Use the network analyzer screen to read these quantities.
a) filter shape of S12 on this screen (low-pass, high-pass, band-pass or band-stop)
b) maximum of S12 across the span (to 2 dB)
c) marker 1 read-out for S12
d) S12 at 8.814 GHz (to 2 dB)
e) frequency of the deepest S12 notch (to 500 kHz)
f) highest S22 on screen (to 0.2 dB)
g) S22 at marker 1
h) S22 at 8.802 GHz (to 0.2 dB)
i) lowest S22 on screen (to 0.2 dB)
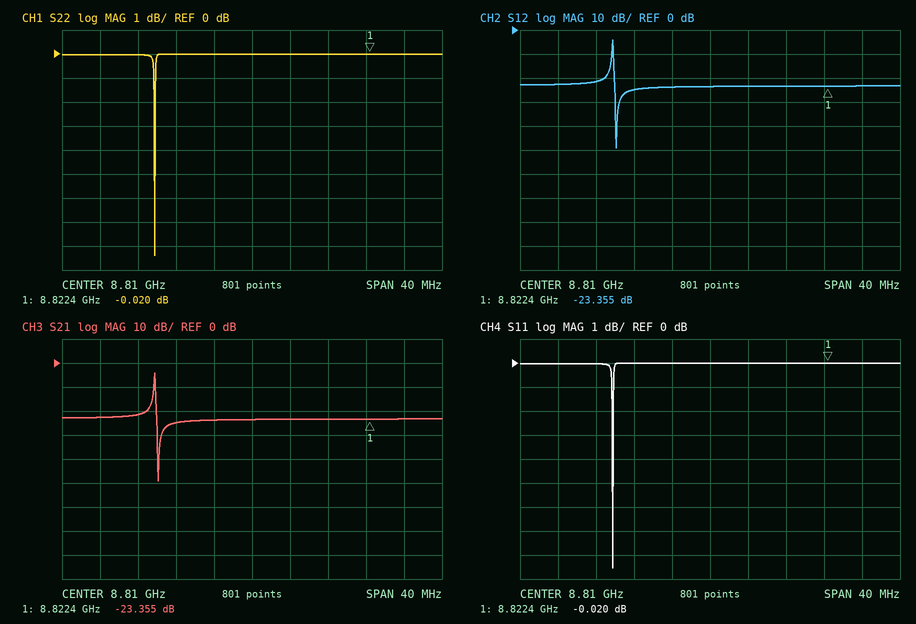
band-pass
-4 dB
-23.355 dB
-24 dB
8.8000 GHz
0.0 dB
-0.020 dB
0.0 dB
-8.4 dB
